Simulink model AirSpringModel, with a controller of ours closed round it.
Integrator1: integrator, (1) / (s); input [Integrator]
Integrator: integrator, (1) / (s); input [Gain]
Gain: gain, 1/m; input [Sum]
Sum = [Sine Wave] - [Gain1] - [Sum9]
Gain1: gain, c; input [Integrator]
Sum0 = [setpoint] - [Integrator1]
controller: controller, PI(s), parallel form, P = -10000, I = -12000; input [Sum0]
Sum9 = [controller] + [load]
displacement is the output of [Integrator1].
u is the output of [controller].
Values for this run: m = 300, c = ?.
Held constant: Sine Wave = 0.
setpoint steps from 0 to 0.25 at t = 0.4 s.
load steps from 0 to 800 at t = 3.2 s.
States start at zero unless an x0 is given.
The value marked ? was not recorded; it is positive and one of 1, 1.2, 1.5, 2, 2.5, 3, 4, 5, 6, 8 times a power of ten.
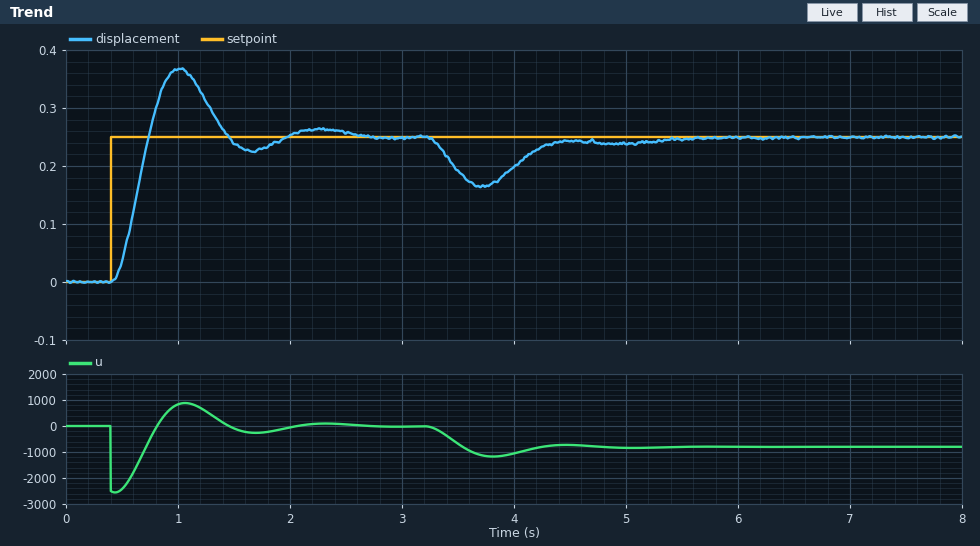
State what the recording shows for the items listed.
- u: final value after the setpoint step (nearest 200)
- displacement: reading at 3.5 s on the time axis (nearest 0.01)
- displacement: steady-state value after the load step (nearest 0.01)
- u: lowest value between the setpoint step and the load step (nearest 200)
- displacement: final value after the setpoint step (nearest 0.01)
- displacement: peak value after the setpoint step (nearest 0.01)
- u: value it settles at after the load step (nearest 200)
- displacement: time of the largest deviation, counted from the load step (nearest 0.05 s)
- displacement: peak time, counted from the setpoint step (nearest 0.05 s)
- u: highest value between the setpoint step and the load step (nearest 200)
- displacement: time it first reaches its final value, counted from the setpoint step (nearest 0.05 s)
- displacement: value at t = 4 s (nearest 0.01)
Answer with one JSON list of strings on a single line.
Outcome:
["0", "0.19", "0.25", "-2600", "0.25", "0.37", "-800", "0.50 s", "0.60 s", "800", "0.35 s", "0.20"]
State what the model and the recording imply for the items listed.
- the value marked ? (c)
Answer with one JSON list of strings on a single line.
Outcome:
["1500"]
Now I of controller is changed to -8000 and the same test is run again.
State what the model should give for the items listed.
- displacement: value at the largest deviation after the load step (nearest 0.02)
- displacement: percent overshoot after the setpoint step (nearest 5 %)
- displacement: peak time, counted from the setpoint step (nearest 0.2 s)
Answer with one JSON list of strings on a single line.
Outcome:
["0.16", "40 %", "0.6 s"]
